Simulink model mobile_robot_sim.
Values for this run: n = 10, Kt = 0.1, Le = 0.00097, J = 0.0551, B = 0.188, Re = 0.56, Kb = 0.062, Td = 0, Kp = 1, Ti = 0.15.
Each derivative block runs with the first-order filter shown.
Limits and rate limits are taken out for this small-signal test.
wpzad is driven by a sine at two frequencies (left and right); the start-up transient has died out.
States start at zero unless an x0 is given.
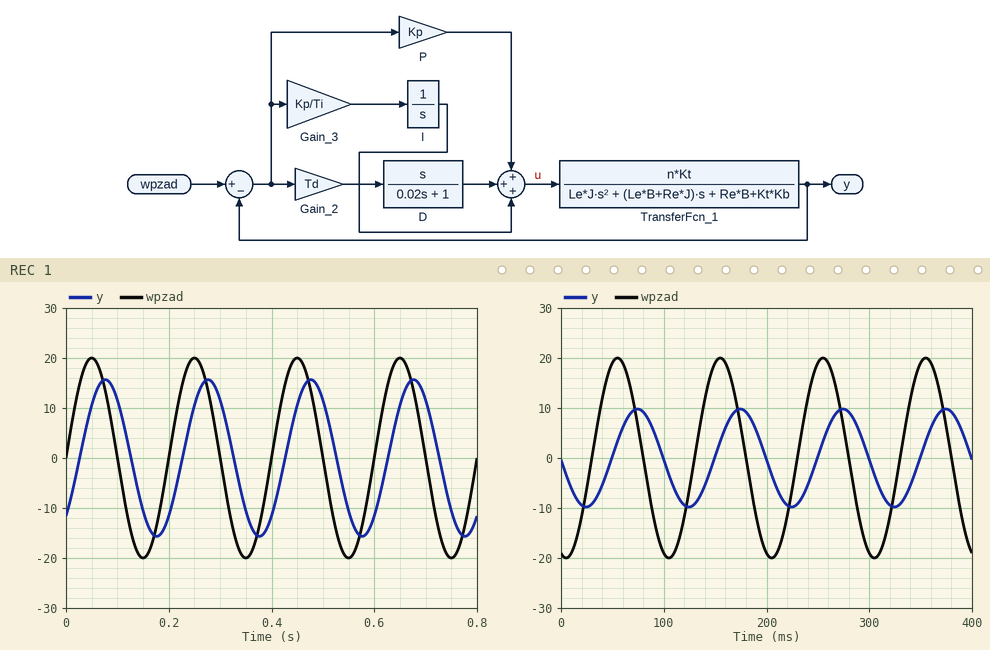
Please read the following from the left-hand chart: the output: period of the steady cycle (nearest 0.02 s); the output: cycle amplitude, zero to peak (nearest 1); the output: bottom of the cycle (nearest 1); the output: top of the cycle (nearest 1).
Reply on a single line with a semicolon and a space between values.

0.20 s; 16; -16; 16
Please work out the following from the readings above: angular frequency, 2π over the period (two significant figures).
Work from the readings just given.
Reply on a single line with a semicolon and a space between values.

31 rad/s
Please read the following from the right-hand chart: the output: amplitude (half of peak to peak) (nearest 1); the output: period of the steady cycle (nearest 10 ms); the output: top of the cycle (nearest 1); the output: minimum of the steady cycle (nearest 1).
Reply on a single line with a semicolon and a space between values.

10; 100 ms; 10; -10
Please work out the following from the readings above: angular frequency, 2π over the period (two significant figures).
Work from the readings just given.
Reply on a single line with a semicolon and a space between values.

0.063 rad/ms
